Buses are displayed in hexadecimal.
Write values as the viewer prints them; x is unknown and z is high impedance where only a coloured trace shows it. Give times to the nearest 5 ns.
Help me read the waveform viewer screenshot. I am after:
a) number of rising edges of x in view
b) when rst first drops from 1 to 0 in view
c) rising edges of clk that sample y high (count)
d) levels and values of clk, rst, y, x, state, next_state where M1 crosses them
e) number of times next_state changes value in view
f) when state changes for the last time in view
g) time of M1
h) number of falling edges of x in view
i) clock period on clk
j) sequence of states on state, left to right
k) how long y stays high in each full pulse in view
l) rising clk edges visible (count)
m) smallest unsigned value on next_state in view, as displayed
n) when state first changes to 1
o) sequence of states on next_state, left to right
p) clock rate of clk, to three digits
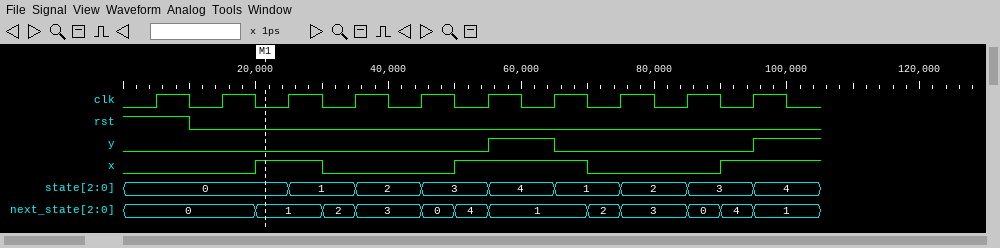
3
10 ns
1
clk=0, rst=0, y=0, x=1, state=0, next_state=1
11
95 ns
20 ns
2
10 ns
0, 1, 2, 3, 4, 1, 2, 3, 4
10 ns
10
0
25 ns
0, 1, 2, 3, 0, 4, 1, 2, 3, 0, 4, 1
100 MHz
